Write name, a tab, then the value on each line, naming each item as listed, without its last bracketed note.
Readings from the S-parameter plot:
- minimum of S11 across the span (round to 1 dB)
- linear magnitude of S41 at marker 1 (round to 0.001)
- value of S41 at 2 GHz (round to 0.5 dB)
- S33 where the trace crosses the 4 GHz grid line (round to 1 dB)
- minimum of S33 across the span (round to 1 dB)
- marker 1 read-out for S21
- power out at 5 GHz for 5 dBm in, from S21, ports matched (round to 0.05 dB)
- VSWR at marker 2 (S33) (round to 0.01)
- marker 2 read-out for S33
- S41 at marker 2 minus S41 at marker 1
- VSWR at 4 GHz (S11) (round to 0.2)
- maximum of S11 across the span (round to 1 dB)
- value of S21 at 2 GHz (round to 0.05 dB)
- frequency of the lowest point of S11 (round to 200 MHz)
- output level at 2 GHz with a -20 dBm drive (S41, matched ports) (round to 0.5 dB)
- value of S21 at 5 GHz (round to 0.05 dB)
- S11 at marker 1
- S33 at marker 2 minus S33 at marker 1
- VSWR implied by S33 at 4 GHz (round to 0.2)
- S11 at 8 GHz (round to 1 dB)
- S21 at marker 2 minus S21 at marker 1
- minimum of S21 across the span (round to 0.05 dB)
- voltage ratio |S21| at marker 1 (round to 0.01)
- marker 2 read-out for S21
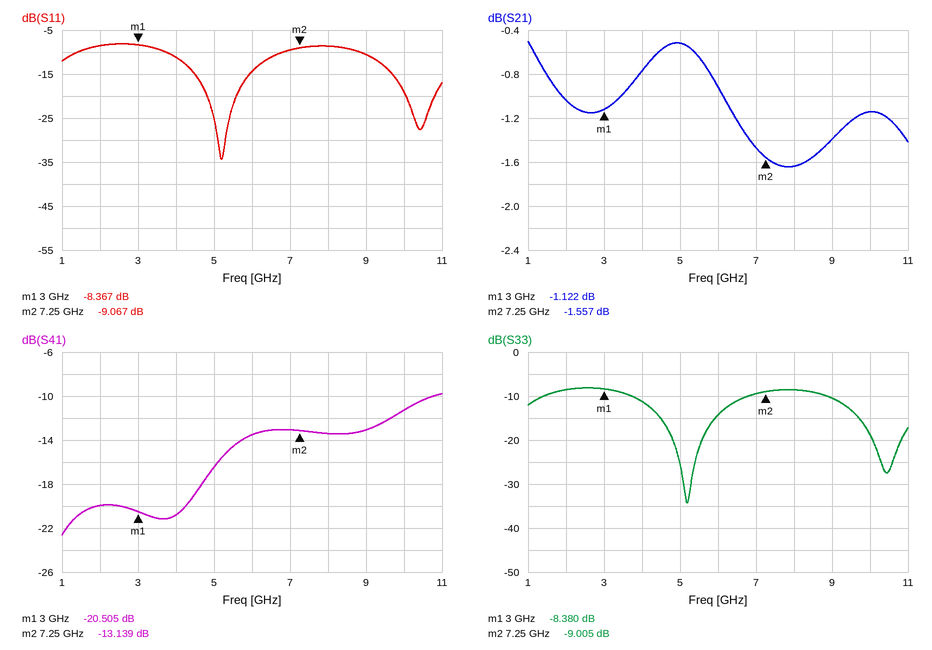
minimum of S11 across the span	-34 dB
linear magnitude of S41 at marker 1	0.094
value of S41 at 2 GHz	-20.0 dB
S33 where the trace crosses the 4 GHz grid line	-11 dB
minimum of S33 across the span	-34 dB
marker 1 read-out for S21	-1.122 dB
power out at 5 GHz for 5 dBm in, from S21, ports matched	4.50 dBm
VSWR at marker 2 (S33)	2.10
marker 2 read-out for S33	-9.005 dB
S41 at marker 2 minus S41 at marker 1	7.366 dB
VSWR at 4 GHz (S11)	1.8
maximum of S11 across the span	-8 dB
value of S21 at 2 GHz	-1.05 dB
frequency of the lowest point of S11	5.2 GHz
output level at 2 GHz with a -20 dBm drive (S41, matched ports)	-40.0 dBm
value of S21 at 5 GHz	-0.50 dB
S11 at marker 1	-8.367 dB
S33 at marker 2 minus S33 at marker 1	-0.625 dB
VSWR implied by S33 at 4 GHz	1.8
S11 at 8 GHz	-9 dB
S21 at marker 2 minus S21 at marker 1	-0.435 dB
minimum of S21 across the span	-1.65 dB
voltage ratio |S21| at marker 1	0.88
marker 2 read-out for S21	-1.557 dB
